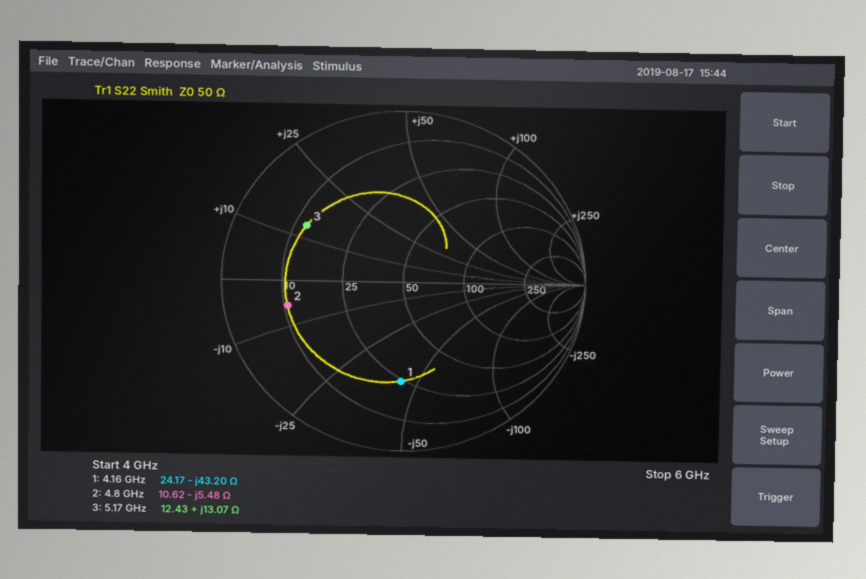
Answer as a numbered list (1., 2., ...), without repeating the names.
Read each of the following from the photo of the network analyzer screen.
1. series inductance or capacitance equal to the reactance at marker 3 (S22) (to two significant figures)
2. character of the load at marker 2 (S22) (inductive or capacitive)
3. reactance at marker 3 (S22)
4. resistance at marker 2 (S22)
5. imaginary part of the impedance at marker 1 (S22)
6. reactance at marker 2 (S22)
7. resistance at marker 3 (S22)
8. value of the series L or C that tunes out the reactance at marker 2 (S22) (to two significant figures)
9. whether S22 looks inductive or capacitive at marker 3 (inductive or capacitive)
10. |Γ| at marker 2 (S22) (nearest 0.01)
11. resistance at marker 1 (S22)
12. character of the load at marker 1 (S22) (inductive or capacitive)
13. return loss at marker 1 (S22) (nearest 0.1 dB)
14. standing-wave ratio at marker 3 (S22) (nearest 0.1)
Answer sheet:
1. 400 pH
2. capacitive
3. +13.07 Ω
4. 10.62 Ω
5. -43.20 Ω
6. -5.48 Ω
7. 12.43 Ω
8. 180 pH
9. inductive
10. 0.65
11. 24.17 Ω
12. capacitive
13. 4.6 dB
14. 4.3
